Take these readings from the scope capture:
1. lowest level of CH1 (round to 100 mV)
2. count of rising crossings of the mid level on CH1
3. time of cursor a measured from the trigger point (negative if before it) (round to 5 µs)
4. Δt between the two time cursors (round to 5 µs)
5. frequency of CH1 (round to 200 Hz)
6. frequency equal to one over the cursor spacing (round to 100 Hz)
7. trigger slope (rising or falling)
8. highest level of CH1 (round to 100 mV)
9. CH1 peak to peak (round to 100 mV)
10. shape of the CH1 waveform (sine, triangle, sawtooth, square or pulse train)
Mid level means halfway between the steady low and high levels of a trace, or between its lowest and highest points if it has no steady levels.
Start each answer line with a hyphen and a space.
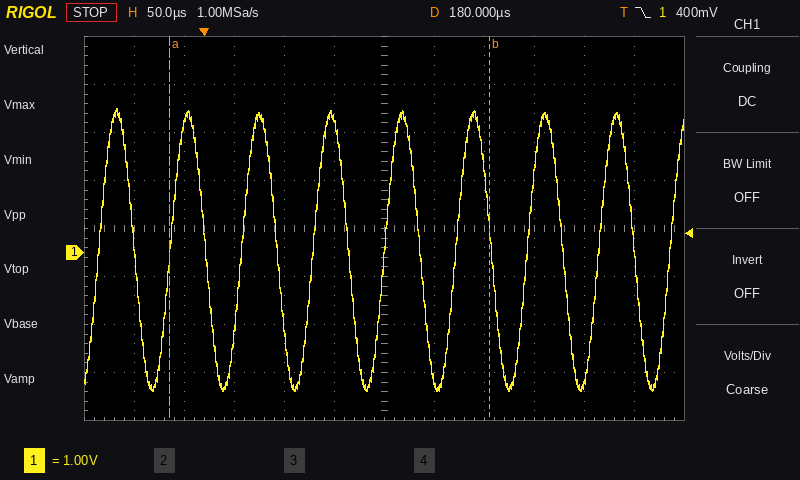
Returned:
- -2.9 V
- 9
- -35 µs
- 320 µs
- 14.0 kHz
- 3.1 kHz
- falling
- 3.0 V
- 5.9 V
- sine
